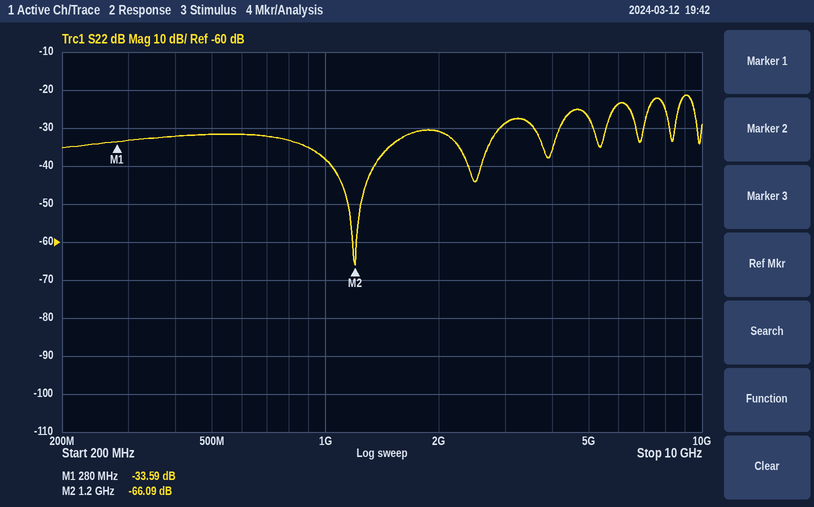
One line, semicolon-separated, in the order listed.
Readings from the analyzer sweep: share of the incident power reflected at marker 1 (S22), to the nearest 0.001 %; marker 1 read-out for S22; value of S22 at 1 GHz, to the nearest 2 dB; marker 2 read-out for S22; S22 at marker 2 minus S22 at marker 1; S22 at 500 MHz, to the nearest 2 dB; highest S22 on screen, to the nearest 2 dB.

0.044 %; -33.59 dB; -38 dB; -66.09 dB; -32.50 dB; -32 dB; -22 dB
